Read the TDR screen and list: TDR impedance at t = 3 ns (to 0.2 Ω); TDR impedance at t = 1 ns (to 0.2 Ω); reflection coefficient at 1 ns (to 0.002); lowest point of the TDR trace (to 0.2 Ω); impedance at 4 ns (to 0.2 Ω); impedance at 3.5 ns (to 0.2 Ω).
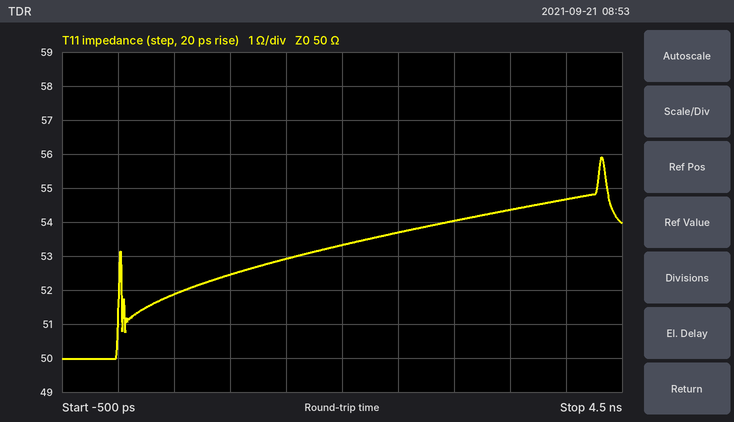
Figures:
54.0 Ω
52.4 Ω
+0.024
50.0 Ω
54.6 Ω
54.4 Ω
